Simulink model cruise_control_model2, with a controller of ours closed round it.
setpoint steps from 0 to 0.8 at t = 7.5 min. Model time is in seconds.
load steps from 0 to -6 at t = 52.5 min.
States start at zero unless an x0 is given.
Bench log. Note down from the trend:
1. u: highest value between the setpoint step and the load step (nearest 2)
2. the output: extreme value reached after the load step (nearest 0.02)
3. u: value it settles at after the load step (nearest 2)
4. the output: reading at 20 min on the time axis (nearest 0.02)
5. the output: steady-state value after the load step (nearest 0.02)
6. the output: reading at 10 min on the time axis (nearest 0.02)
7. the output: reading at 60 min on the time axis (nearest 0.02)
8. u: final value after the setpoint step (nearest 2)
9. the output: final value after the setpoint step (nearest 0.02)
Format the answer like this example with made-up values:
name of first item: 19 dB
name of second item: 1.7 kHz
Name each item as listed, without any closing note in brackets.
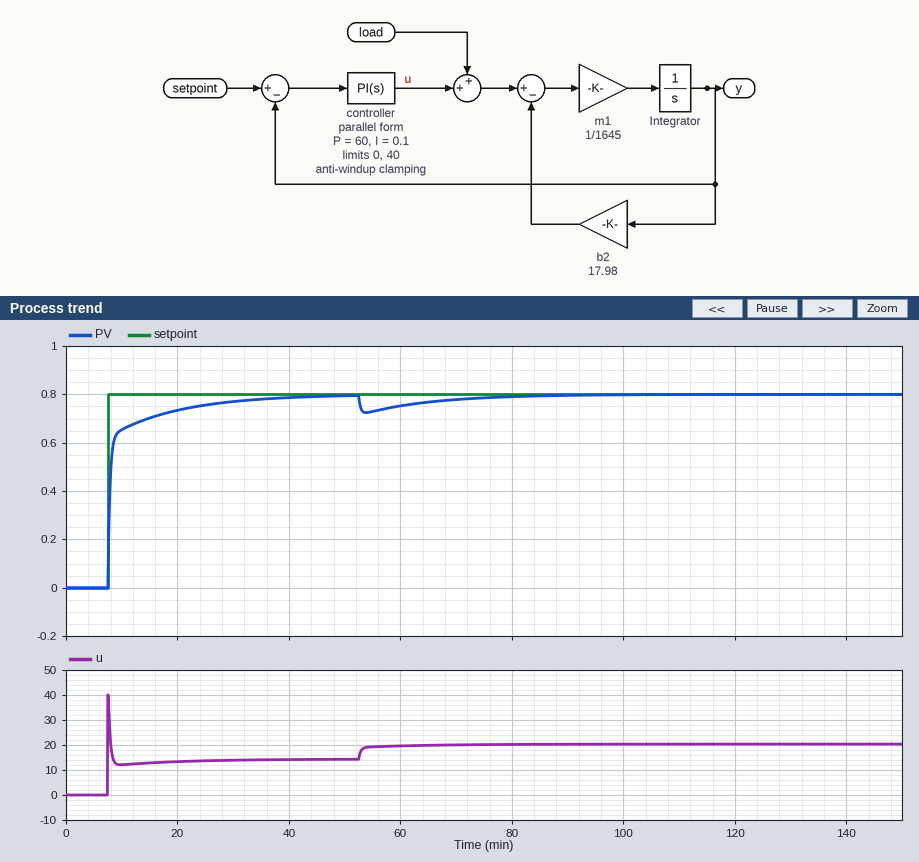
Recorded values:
u: highest value between the setpoint step and the load step: 40
the output: extreme value reached after the load step: 0.72
u: value it settles at after the load step: 20
the output: reading at 20 min on the time axis: 0.74
the output: steady-state value after the load step: 0.80
the output: reading at 10 min on the time axis: 0.66
the output: reading at 60 min on the time axis: 0.76
u: final value after the setpoint step: 14
the output: final value after the setpoint step: 0.80
